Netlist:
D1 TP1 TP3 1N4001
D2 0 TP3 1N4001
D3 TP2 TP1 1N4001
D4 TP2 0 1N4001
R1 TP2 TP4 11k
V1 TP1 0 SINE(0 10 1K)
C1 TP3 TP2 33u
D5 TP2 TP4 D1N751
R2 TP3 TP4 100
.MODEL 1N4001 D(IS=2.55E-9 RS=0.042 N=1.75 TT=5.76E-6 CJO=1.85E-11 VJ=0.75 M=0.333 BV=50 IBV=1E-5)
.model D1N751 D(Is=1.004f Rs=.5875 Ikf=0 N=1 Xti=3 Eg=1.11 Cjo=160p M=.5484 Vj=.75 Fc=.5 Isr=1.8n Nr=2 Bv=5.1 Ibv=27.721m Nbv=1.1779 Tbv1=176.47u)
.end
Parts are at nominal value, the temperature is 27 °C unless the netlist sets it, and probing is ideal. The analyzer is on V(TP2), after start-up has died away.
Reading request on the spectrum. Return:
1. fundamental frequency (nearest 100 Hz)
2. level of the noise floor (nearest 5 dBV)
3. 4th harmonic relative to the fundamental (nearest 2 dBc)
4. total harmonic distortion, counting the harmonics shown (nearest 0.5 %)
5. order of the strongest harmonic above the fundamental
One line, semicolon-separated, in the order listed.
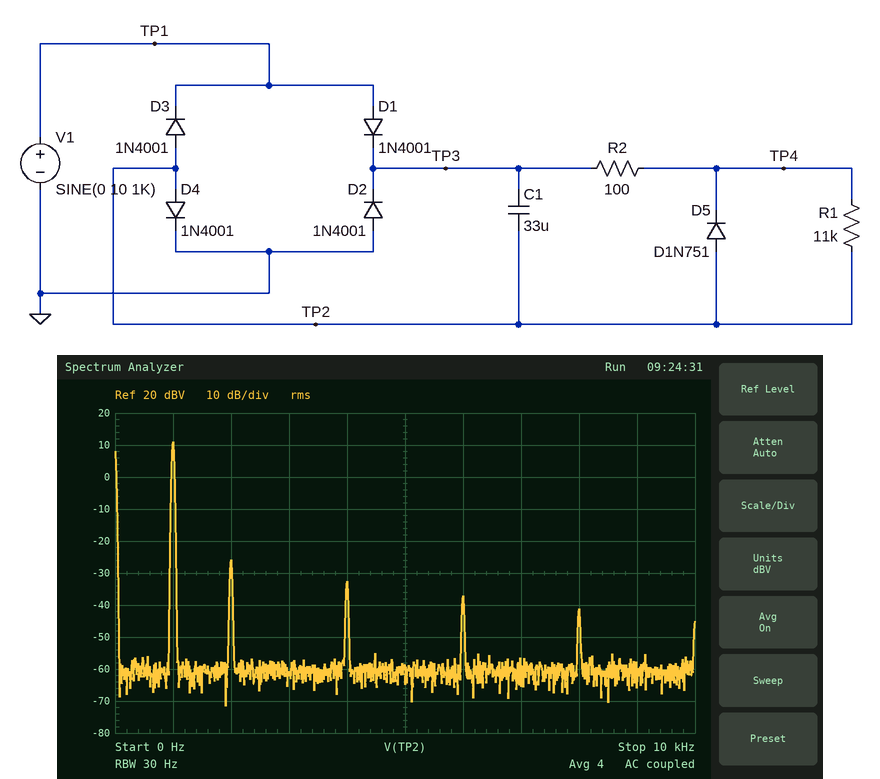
1.0 kHz; -60 dBV; -44 dBc; 1.5 %; 2
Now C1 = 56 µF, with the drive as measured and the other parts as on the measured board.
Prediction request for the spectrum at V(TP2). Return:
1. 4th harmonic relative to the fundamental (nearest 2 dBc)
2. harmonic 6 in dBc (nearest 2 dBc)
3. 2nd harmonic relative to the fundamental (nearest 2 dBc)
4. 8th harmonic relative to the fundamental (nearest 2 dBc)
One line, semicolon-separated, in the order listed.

-48 dBc; -52 dBc; -42 dBc; -56 dBc
